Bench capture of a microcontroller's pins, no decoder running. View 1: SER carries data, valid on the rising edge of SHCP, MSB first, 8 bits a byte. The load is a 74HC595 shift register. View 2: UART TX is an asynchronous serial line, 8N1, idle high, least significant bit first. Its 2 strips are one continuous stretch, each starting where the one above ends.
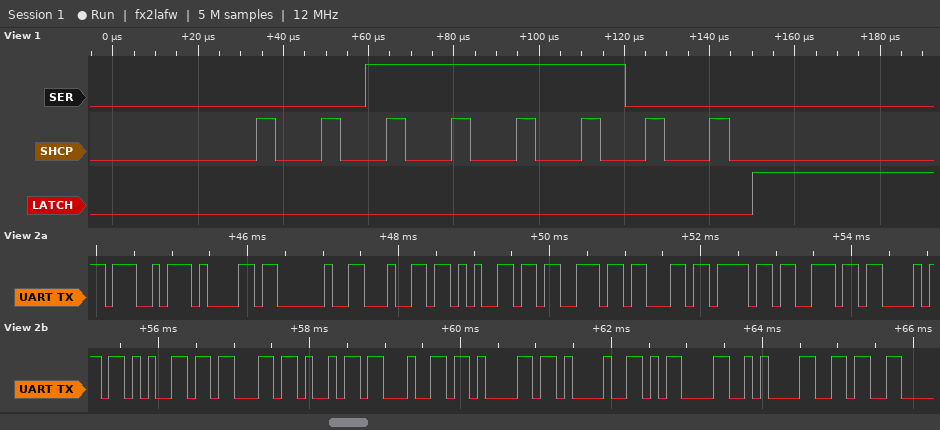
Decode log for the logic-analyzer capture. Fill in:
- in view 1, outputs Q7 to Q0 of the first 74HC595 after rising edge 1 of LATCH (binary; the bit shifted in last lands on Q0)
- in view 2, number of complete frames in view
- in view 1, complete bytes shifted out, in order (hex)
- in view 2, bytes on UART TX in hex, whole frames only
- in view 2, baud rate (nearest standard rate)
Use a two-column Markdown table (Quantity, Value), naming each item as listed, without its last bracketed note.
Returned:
| Quantity | Value |
|---|---|
| in view 1, outputs Q7 to Q0 of the first 74HC595 after rising edge 1 of LATCH | 00111100 |
| in view 2, number of complete frames in view | 19 |
| in view 1, complete bytes shifted out, in order | 3C |
| in view 2, bytes on UART TX in hex, whole frames only | A7 61 20 64 65 73 63 6F 6E 68 65 63 69 64 61 21 0D 0A 36 |
| in view 2, baud rate | 9600 baud |
